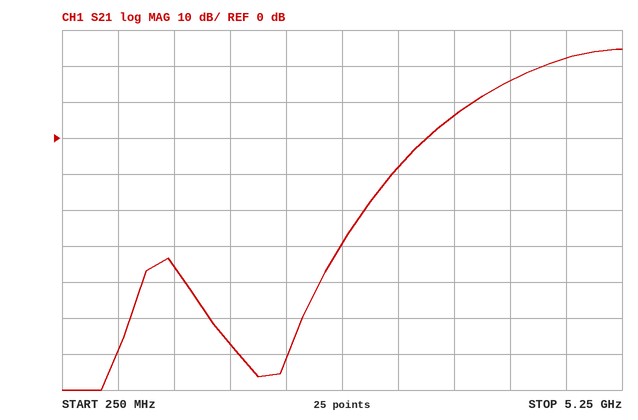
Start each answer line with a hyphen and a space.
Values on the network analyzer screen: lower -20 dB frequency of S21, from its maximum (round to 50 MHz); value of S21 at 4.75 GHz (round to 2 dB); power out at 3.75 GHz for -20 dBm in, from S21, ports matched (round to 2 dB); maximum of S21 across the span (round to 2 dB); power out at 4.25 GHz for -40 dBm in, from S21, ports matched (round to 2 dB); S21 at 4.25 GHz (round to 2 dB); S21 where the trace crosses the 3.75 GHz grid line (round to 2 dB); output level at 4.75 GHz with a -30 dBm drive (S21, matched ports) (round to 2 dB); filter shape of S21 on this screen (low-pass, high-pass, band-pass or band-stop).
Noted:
- 3.70 GHz
- 22 dB
- -14 dBm
- 24 dB
- -24 dBm
- 16 dB
- 6 dB
- -8 dBm
- high-pass
